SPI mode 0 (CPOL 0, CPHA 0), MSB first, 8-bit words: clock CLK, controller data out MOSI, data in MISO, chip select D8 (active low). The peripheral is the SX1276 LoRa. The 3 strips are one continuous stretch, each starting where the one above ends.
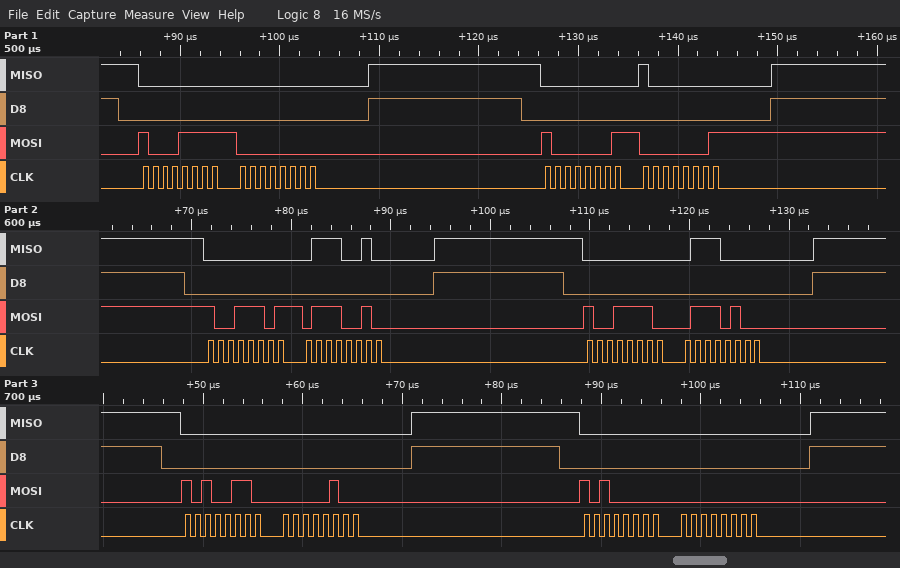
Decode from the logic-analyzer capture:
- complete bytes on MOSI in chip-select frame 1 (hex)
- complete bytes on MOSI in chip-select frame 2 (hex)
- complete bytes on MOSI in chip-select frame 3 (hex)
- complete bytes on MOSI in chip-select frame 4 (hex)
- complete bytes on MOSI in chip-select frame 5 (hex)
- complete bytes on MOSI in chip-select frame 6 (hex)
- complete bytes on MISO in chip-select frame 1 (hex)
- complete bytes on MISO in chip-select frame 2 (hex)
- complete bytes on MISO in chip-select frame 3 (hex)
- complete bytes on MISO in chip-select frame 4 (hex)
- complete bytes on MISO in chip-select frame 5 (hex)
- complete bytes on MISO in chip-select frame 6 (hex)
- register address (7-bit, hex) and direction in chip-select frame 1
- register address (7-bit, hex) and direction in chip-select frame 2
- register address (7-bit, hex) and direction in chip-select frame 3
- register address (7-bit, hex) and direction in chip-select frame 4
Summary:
0x8F 0x00
0x81 0x01
0x9D 0x72
0x9E 0x74
0xA6 0x04
0xA0 0x00
0x00 0x00
0x00 0x80
0x00 0x72
0x00 0x70
0x00 0x00
0x00 0x00
0x0F write
0x01 write
0x1D write
0x1E write
